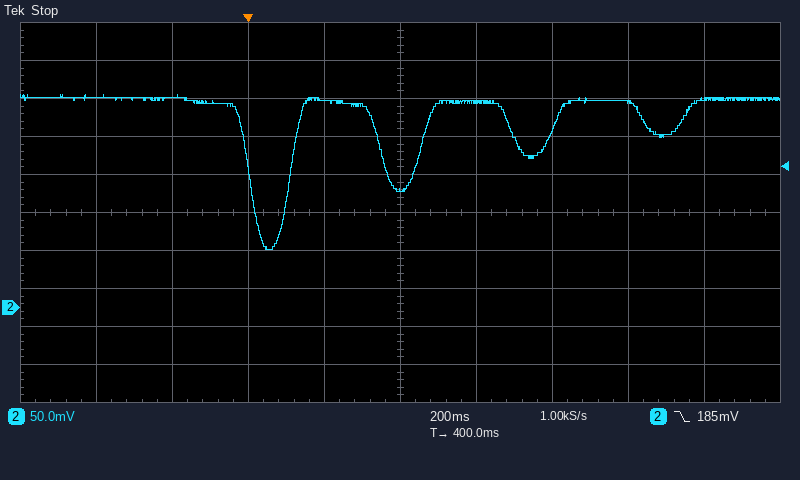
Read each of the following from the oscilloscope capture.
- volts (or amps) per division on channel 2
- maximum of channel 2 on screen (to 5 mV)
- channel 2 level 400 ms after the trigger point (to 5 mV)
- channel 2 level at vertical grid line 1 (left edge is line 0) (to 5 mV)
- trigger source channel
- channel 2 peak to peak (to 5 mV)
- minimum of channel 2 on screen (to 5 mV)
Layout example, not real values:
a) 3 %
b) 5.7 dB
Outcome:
a) 50 mV
b) 280 mV
c) 155 mV
d) 275 mV
e) channel 2
f) 205 mV
g) 75 mV
